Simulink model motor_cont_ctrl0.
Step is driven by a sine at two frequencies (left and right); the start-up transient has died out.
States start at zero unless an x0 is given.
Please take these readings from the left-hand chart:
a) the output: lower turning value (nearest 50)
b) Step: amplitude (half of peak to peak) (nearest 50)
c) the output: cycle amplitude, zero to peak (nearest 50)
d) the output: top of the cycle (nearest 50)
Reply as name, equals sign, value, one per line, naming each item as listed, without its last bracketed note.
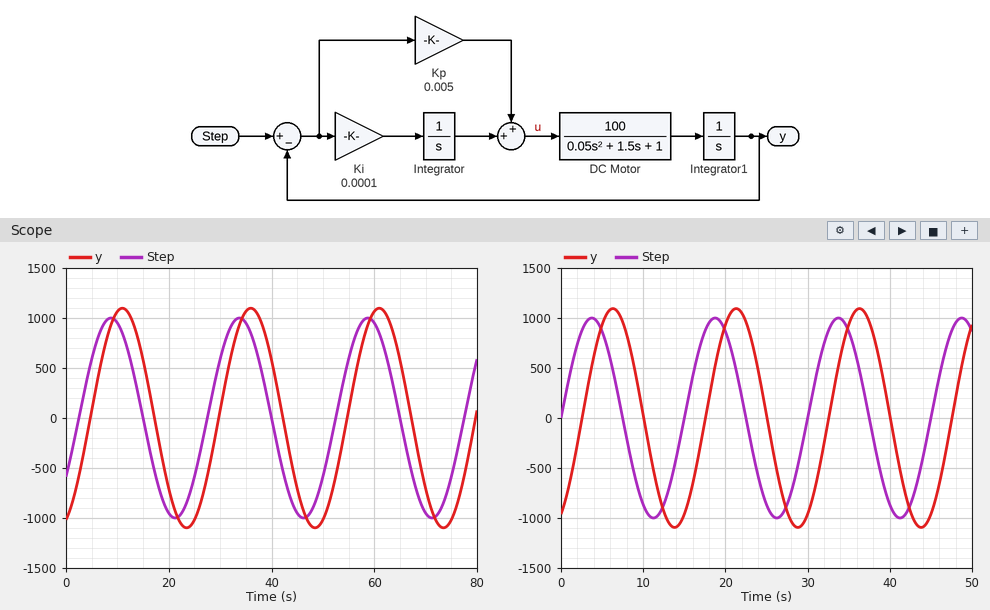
the output: lower turning value = -1100
Step: amplitude (half of peak to peak) = 1000
the output: cycle amplitude, zero to peak = 1100
the output: top of the cycle = 1100
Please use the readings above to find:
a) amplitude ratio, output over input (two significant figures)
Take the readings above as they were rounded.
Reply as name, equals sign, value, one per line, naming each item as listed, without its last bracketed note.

amplitude ratio, output over input = 1.1
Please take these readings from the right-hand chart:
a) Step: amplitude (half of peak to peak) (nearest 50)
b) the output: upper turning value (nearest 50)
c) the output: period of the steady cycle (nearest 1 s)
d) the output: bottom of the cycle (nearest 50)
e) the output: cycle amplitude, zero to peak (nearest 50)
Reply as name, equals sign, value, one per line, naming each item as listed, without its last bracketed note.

Step: amplitude (half of peak to peak) = 1000
the output: upper turning value = 1100
the output: period of the steady cycle = 15 s
the output: bottom of the cycle = -1100
the output: cycle amplitude, zero to peak = 1100
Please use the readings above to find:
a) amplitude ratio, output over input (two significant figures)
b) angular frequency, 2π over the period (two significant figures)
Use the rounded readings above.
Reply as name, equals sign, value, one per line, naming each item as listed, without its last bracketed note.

amplitude ratio, output over input = 1.1
angular frequency, 2π over the period = 0.42 rad/s
